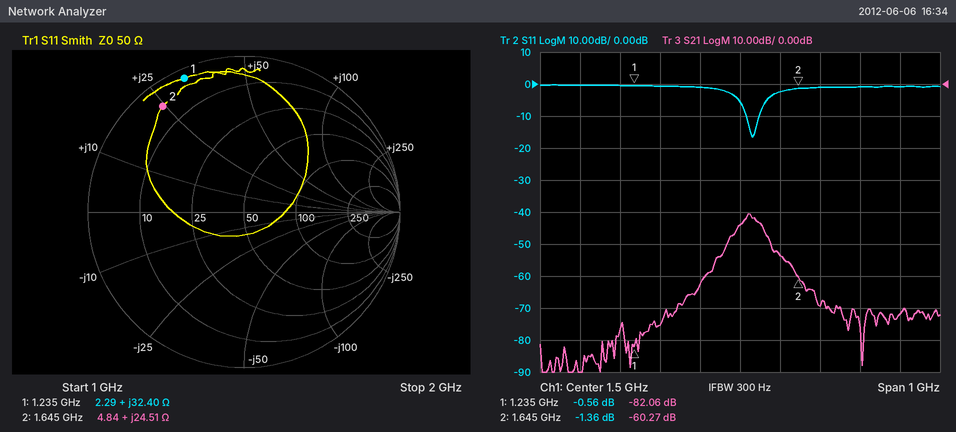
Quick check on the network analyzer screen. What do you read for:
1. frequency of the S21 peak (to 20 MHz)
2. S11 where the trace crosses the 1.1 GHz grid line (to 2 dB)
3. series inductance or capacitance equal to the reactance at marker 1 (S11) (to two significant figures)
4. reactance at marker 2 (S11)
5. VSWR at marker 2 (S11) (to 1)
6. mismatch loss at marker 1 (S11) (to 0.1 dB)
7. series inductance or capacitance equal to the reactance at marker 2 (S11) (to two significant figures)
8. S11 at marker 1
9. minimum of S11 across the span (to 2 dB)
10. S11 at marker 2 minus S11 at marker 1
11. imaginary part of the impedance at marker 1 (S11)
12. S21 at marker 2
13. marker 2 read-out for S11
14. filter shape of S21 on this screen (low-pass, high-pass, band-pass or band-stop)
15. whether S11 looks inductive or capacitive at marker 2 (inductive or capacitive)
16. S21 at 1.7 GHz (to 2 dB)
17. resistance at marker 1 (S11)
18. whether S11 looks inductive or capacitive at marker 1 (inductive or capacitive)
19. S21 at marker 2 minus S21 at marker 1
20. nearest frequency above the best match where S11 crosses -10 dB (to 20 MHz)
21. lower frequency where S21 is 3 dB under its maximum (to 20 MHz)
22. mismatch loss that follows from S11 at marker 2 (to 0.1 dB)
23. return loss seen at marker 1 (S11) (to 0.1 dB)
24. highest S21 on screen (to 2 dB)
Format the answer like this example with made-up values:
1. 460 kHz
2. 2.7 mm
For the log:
1. 1.52 GHz
2. 0 dB
3. 4.2 nH
4. +24.51 Ω
5. 13
6. 9.2 dB
7. 2.4 nH
8. -0.56 dB
9. -16 dB
10. -0.80 dB
11. +32.40 Ω
12. -60.27 dB
13. -1.36 dB
14. band-pass
15. inductive
16. -70 dB
17. 2.29 Ω
18. inductive
19. 21.79 dB
20. 1.54 GHz
21. 1.50 GHz
22. 5.7 dB
23. 0.6 dB
24. -40 dB
